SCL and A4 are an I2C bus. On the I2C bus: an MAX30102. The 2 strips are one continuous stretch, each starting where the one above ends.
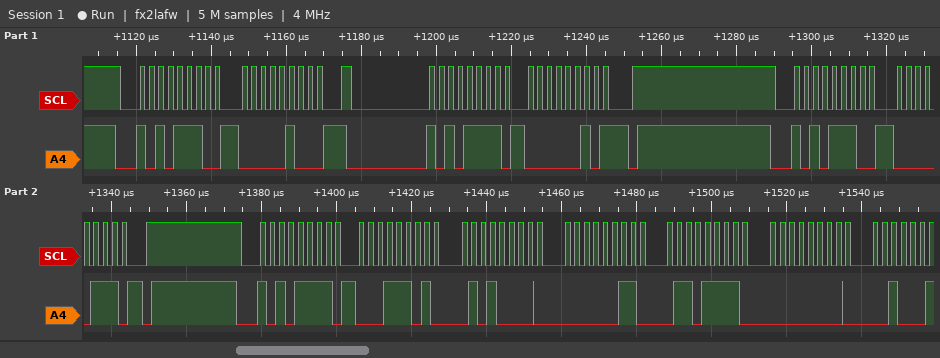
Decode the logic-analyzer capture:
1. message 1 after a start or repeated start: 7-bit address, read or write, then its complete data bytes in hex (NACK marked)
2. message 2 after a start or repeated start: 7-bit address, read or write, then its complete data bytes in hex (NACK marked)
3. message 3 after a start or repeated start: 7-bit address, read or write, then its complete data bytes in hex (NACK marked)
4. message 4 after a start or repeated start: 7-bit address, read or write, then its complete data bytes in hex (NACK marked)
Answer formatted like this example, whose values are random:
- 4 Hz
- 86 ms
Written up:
- 0x57 write: 04
- 0x57 read: 02 NACK
- 0x57 write: 07
- 0x57 read: 1D 50 03 6F 00
